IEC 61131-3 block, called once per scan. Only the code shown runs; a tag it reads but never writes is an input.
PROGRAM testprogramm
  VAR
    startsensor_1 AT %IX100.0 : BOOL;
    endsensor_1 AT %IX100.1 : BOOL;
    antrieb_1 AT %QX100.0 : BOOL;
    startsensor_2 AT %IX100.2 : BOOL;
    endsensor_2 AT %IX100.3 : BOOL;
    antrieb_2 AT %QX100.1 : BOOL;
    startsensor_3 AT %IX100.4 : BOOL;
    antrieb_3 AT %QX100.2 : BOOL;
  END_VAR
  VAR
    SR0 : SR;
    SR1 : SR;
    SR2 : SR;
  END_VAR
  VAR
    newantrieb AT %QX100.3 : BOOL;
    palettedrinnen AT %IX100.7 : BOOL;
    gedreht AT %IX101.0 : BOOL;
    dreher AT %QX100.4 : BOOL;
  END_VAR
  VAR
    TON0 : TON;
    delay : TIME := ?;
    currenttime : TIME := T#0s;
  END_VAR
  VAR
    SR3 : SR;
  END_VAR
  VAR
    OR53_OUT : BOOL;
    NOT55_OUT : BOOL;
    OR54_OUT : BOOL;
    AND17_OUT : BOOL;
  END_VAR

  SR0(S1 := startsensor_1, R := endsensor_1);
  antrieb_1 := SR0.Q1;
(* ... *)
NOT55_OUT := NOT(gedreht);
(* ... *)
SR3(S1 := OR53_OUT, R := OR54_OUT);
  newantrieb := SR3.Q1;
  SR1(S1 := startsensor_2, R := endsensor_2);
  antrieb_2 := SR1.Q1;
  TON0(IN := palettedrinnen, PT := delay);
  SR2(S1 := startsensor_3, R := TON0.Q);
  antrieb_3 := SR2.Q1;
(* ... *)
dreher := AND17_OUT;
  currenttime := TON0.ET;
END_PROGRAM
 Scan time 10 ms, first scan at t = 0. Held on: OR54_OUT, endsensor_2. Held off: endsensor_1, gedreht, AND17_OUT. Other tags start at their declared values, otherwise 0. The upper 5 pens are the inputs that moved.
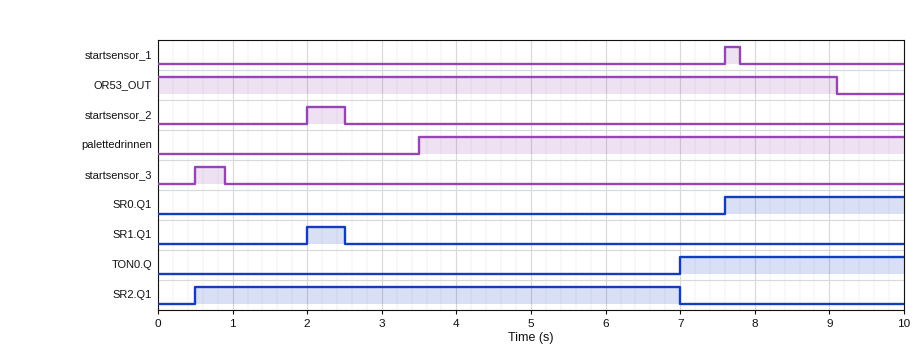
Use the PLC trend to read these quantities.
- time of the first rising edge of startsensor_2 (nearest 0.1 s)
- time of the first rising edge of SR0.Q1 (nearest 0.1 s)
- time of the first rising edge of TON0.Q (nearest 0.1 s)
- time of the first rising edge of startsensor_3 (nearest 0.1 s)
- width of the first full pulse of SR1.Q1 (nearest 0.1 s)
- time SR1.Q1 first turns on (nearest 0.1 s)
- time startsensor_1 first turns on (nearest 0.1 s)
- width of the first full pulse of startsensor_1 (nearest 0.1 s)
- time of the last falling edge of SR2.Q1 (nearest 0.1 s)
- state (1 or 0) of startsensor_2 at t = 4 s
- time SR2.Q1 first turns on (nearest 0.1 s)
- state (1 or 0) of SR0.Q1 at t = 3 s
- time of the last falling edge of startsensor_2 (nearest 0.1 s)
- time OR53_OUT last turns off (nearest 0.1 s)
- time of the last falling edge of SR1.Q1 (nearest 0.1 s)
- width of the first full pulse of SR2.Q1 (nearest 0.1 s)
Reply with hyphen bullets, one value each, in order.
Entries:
- 2.0 s
- 7.6 s
- 7.0 s
- 0.5 s
- 0.5 s
- 2.0 s
- 7.6 s
- 0.2 s
- 7.0 s
- 0
- 0.5 s
- 0
- 2.5 s
- 9.1 s
- 2.5 s
- 6.5 s
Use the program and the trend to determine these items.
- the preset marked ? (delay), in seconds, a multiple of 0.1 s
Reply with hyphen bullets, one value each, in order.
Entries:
- 3.5 s
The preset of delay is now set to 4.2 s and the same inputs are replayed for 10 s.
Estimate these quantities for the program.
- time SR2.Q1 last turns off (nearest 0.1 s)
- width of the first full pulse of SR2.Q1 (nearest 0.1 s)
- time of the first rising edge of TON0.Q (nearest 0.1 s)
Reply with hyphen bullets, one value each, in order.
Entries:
- 7.7 s
- 7.2 s
- 7.7 s
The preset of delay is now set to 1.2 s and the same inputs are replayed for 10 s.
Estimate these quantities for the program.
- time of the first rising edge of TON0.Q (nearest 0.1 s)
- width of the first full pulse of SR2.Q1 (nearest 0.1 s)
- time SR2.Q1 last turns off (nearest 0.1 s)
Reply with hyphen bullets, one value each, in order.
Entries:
- 4.7 s
- 4.2 s
- 4.7 s
